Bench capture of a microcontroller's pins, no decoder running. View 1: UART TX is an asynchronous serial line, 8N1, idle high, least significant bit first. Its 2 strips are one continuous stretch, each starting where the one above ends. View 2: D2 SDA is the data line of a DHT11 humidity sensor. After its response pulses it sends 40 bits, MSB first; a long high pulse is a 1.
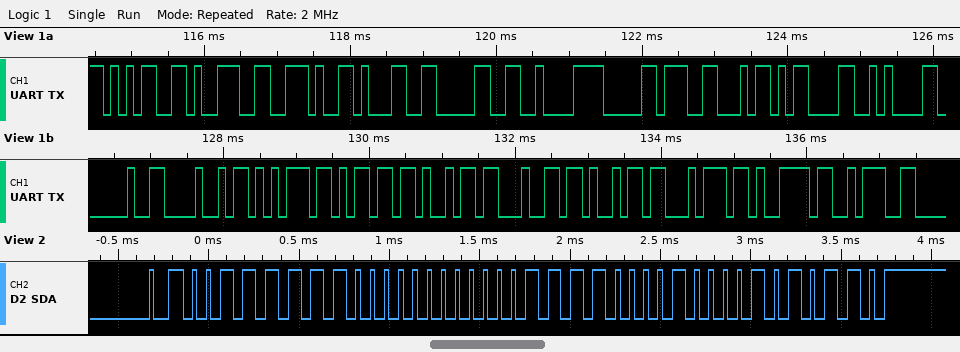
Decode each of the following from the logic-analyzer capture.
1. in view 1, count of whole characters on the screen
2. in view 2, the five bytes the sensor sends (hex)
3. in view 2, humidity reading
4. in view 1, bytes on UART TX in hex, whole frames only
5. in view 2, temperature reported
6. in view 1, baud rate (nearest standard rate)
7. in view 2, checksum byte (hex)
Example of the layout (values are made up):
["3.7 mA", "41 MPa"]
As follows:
["20", "3F 00 0F 08 56", "63 %", "35 39 2E 31 30 C2 B0 46 0D 0A 20 48 75 6D 69 64 69 74 79 3A", "15.8 °C", "9600 baud", "0x56"]
